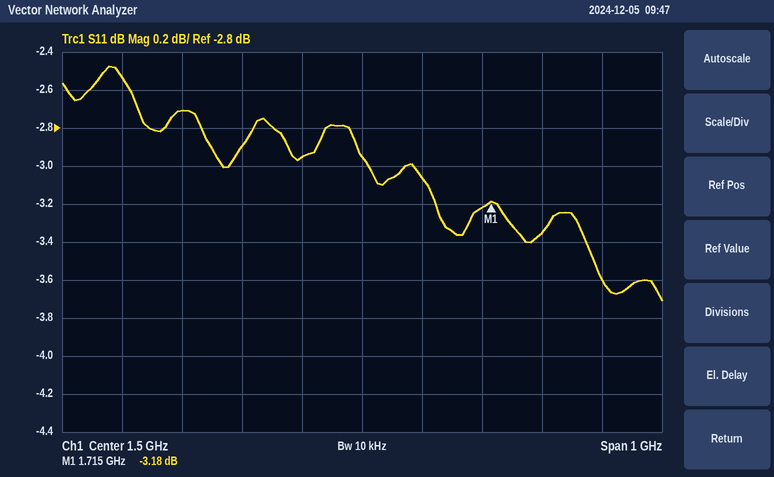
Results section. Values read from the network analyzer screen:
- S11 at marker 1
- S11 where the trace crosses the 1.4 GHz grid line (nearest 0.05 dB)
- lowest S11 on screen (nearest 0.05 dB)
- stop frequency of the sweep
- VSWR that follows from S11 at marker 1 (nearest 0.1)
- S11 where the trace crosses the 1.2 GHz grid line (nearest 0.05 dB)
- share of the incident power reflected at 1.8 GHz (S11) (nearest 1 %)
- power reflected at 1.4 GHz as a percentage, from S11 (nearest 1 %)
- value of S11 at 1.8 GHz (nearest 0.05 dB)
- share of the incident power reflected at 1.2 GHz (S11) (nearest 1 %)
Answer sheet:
-3.18 dB
-2.95 dB
-3.70 dB
2 GHz
5.5
-2.70 dB
46 %
51 %
-3.35 dB
54 %
